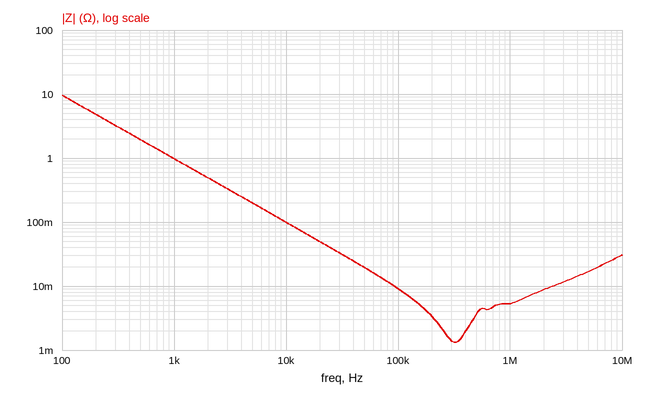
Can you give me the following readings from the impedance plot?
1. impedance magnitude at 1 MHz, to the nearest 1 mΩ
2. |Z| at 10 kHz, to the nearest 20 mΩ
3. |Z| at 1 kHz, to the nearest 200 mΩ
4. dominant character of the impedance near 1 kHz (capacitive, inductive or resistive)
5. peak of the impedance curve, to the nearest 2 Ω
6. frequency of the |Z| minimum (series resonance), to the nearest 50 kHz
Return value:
5 mΩ
100 mΩ
1.0 Ω
capacitive
10 Ω
300 kHz
